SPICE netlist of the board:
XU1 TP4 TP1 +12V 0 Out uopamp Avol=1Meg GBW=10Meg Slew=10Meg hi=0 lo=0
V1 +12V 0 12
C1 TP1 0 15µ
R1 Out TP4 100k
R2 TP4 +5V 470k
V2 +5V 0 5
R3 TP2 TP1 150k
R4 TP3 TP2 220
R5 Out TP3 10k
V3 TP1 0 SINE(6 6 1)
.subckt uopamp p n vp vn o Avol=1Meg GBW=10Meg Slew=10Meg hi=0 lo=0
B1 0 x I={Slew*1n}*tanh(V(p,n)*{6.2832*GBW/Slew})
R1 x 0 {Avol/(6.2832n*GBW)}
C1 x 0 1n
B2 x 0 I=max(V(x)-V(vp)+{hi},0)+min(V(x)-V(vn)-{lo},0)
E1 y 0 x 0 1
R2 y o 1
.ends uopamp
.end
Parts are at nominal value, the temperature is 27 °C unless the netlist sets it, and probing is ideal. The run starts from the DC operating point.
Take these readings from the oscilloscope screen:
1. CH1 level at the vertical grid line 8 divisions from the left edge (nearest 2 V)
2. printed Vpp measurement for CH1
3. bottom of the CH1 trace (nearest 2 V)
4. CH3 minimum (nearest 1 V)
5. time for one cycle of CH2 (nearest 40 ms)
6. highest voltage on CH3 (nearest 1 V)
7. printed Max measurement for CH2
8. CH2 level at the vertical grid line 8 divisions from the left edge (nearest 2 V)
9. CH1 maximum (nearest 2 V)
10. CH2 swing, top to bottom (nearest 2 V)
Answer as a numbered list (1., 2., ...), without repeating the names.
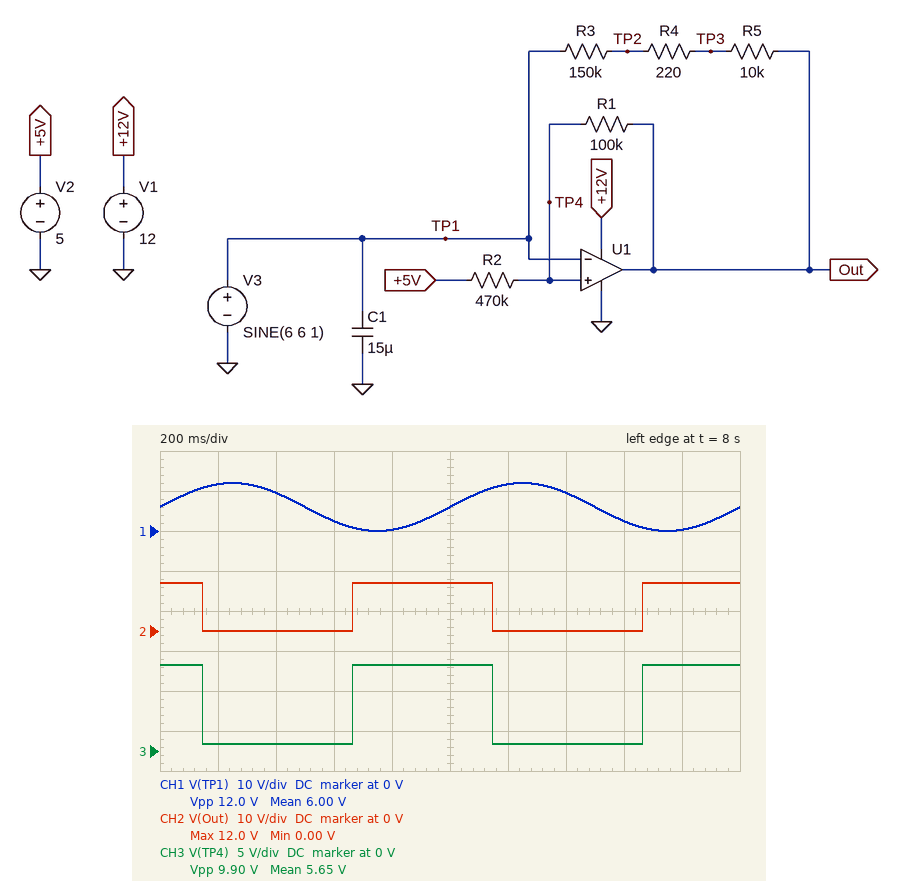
1. 2 V
2. 12.0 V
3. 0 V
4. 1 V
5. 1.00 s
6. 11 V
7. 12.0 V
8. 0 V
9. 12 V
10. 12 V
